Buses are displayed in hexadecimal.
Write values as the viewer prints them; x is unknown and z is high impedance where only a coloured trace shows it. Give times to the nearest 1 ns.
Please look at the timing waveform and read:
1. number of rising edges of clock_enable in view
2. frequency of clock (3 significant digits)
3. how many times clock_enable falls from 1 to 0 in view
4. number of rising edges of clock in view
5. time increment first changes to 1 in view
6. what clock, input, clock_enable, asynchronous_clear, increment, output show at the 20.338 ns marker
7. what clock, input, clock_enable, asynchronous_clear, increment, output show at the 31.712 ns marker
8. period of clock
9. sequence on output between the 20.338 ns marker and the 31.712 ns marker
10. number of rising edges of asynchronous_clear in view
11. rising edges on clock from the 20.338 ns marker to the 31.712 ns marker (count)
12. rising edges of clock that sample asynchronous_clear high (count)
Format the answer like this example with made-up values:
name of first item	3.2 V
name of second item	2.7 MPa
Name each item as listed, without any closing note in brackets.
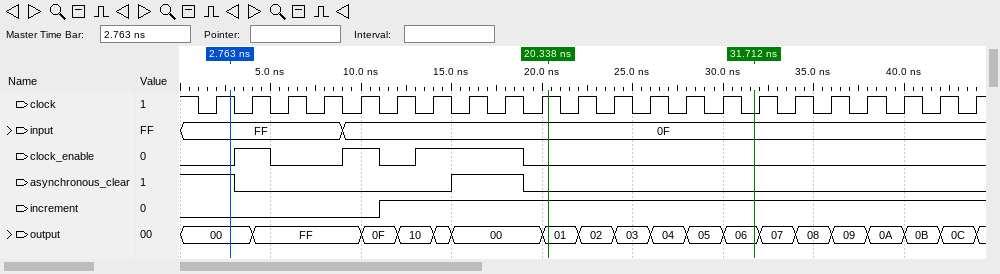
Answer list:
number of rising edges of clock_enable in view	3
frequency of clock	500 MHz
how many times clock_enable falls from 1 to 0 in view	3
number of rising edges of clock in view	22
time increment first changes to 1 in view	11 ns
what clock, input, clock_enable, asynchronous_clear, increment, output show at the 20.338 ns marker	clock=1, input=0F, clock_enable=0, asynchronous_clear=0, increment=1, output=01
what clock, input, clock_enable, asynchronous_clear, increment, output show at the 31.712 ns marker	clock=0, input=0F, clock_enable=0, asynchronous_clear=0, increment=1, output=06
period of clock	2 ns
sequence on output between the 20.338 ns marker and the 31.712 ns marker	01, 02, 03, 04, 05, 06
number of rising edges of asynchronous_clear in view	1
rising edges on clock from the 20.338 ns marker to the 31.712 ns marker	5
rising edges of clock that sample asynchronous_clear high	3
